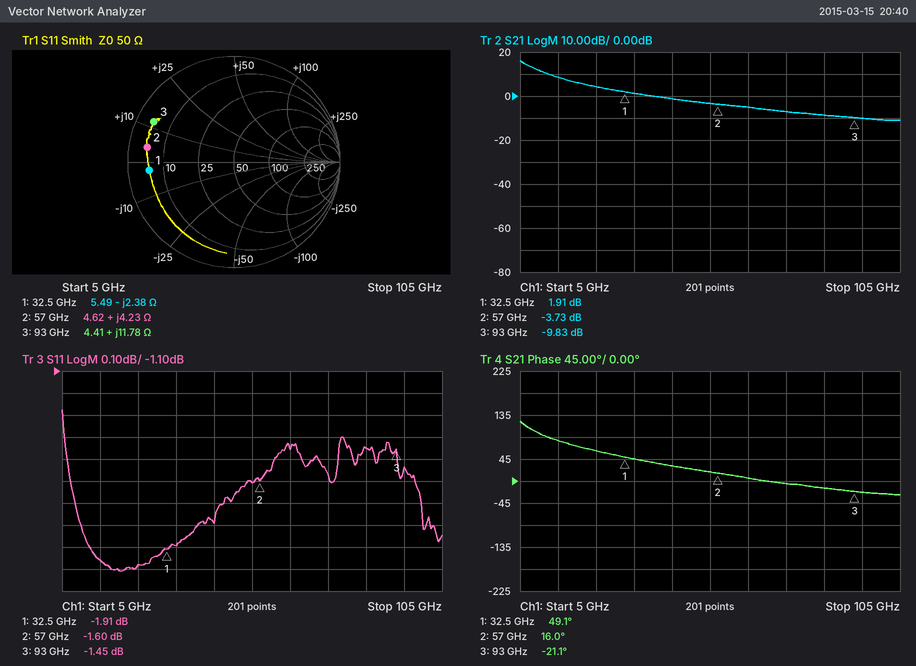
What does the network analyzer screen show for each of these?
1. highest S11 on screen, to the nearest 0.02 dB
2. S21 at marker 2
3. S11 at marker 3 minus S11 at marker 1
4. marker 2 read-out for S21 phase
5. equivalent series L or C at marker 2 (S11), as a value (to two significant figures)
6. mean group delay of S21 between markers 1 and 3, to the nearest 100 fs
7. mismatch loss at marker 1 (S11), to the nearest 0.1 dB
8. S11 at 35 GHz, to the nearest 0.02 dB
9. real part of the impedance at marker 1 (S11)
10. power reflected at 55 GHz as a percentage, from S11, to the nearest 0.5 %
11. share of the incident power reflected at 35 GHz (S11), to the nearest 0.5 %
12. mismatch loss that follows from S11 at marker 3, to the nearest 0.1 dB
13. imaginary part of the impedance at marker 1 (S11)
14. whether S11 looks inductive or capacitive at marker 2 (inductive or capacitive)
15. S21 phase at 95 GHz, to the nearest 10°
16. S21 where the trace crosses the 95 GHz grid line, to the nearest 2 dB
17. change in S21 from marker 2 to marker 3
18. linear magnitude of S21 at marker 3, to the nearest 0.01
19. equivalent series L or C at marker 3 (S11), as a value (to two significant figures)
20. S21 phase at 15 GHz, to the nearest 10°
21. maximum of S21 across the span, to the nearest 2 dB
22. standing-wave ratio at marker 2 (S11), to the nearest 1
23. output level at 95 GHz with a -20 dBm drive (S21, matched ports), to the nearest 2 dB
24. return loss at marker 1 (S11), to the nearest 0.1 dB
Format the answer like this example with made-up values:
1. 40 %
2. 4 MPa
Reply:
1. -1.28 dB
2. -3.73 dB
3. 0.46 dB
4. 16.0°
5. 12 pH
6. 3.2 ps
7. 4.5 dB
8. -1.90 dB
9. 5.49 Ω
10. 69.0 %
11. 64.5 %
12. 5.5 dB
13. -2.38 Ω
14. inductive
15. -20°
16. -10 dB
17. -6.10 dB
18. 0.32
19. 20 pH
20. 80°
21. 16 dB
22. 11
23. -30 dBm
24. 1.9 dB
